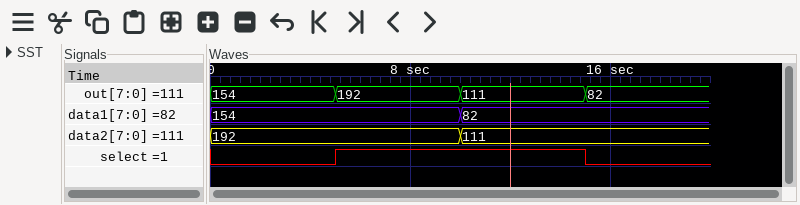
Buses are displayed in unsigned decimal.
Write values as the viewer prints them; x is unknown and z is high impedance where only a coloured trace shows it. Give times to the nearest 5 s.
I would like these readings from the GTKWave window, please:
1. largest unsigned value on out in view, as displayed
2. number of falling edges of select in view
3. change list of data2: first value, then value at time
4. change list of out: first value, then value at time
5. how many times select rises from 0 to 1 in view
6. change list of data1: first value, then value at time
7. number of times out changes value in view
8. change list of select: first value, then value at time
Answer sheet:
192
1
192, 111 at 10 s
154, 192 at 5 s, 111 at 10 s, 82 at 15 s
1
154, 82 at 10 s
3
0, 1 at 5 s, 0 at 15 s
